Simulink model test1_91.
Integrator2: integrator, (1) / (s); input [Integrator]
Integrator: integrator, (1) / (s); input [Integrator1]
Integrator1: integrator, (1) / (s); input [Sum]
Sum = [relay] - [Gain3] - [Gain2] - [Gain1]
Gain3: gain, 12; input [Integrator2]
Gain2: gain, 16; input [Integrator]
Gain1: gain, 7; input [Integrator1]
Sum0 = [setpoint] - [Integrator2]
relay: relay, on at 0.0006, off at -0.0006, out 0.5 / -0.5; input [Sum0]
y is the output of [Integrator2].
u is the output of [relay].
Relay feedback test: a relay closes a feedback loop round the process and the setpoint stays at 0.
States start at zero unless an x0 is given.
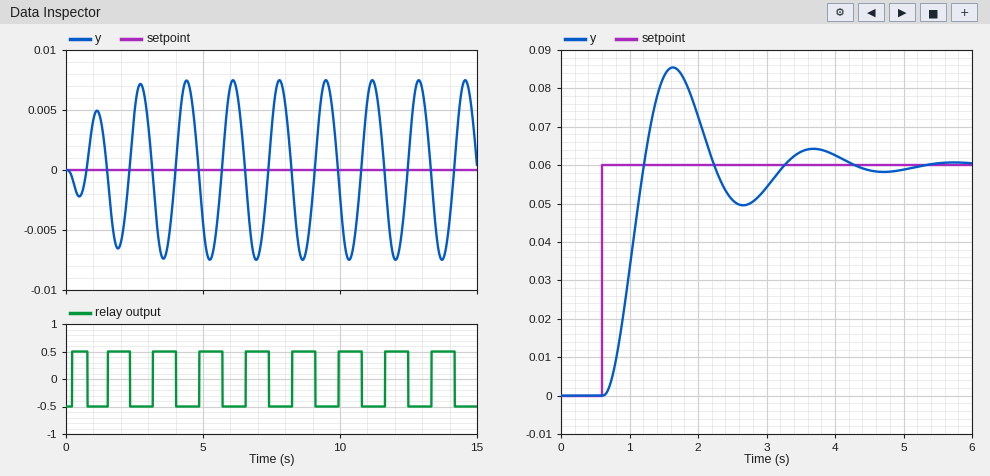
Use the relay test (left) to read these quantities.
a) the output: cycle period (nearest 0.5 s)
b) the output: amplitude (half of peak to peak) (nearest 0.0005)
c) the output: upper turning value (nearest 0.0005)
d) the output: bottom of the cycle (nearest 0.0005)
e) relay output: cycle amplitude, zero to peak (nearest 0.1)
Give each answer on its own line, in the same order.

1.5 s
0.0075
0.0075
-0.0075
0.5
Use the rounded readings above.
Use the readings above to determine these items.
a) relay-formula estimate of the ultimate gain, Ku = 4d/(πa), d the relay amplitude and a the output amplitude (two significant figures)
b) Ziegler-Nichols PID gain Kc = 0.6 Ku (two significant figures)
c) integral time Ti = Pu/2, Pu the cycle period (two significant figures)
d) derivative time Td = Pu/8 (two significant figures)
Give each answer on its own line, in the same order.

85
51
0.75 s
0.19 s
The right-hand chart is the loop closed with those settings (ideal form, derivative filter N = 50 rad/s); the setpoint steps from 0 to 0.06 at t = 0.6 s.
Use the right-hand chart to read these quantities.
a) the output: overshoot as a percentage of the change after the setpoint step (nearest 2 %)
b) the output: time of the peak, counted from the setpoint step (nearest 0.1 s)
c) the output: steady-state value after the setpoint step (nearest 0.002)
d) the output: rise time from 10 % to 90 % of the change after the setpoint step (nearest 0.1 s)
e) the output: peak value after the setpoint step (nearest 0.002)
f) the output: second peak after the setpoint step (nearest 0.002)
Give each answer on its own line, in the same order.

42 %
1.0 s
0.060
0.4 s
0.086
0.064
